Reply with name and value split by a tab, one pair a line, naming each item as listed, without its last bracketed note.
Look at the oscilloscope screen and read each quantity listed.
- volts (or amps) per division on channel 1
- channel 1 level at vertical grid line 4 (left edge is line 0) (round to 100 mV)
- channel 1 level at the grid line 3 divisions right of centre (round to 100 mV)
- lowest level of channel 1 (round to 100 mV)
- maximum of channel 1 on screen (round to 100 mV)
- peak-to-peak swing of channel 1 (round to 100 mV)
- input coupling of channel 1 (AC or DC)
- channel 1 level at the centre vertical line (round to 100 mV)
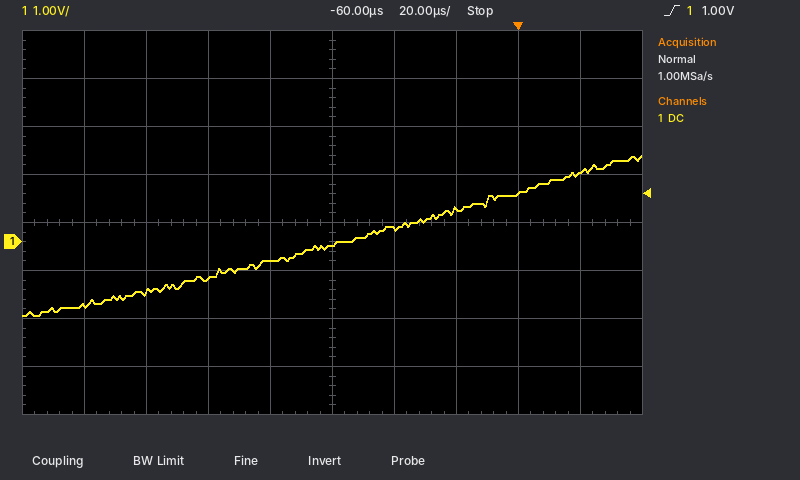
volts (or amps) per division on channel 1	1 V
channel 1 level at vertical grid line 4 (left edge is line 0)	-400 mV
channel 1 level at the grid line 3 divisions right of centre	1.0 V
lowest level of channel 1	-1.5 V
maximum of channel 1 on screen	1.8 V
peak-to-peak swing of channel 1	3.3 V
input coupling of channel 1	DC
channel 1 level at the centre vertical line	-100 mV
